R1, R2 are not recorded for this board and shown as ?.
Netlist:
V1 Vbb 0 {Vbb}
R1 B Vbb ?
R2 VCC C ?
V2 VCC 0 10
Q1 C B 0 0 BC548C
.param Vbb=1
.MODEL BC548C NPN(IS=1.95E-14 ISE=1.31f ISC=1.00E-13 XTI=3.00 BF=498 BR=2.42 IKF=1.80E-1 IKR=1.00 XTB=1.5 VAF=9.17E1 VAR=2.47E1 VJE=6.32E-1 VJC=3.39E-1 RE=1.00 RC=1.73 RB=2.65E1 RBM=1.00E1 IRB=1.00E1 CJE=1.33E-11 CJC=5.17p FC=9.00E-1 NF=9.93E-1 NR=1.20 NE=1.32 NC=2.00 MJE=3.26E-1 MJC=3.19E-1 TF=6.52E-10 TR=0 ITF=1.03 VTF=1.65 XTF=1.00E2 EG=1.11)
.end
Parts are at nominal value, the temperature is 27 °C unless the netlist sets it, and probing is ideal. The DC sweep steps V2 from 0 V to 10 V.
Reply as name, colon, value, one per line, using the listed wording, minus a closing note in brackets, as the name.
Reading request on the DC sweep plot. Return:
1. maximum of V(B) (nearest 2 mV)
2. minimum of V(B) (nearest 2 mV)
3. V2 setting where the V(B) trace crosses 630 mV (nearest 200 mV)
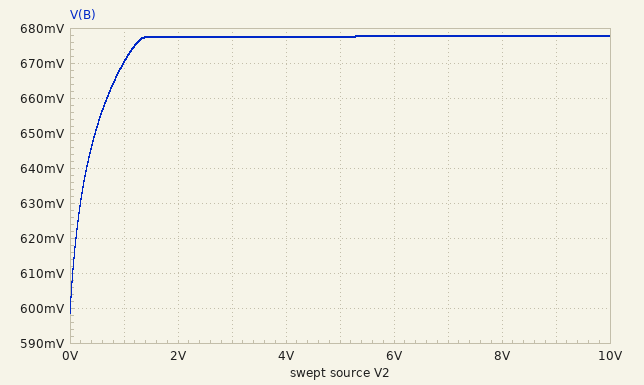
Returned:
maximum of V(B): 678 mV
minimum of V(B): 598 mV
V2 setting where the V(B) trace crosses 630 mV: 200 mV
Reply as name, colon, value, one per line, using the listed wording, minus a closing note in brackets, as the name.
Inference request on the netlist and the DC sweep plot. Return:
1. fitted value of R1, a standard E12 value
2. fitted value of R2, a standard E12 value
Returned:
fitted value of R1, a standard E12 value: 33 kΩ
fitted value of R2, a standard E12 value: 270 Ω
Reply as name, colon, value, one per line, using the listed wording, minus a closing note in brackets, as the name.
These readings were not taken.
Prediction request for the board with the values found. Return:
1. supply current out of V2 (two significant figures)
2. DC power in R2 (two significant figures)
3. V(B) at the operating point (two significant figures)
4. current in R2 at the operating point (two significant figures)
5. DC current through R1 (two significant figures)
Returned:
supply current out of V2: 4.8 mA
DC power in R2: 6.2 mW
V(B) at the operating point: 680 mV
current in R2 at the operating point: 4.8 mA
DC current through R1: 9.8 µA
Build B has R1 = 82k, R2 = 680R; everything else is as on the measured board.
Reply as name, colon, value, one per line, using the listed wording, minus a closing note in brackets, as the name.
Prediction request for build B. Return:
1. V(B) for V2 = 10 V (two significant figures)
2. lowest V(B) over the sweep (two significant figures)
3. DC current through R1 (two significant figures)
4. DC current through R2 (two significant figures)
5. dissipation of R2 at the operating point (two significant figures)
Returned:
V(B) for V2 = 10 V: 650 mV
lowest V(B) over the sweep: 570 mV
DC current through R1: 4.2 µA
DC current through R2: 2.1 mA
dissipation of R2 at the operating point: 2.9 mW
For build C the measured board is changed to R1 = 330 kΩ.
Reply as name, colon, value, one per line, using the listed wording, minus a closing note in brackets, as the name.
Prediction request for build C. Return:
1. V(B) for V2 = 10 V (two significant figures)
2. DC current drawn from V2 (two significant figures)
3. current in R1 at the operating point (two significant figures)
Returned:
V(B) for V2 = 10 V: 620 mV
DC current drawn from V2: 570 µA
current in R1 at the operating point: 1.2 µA
